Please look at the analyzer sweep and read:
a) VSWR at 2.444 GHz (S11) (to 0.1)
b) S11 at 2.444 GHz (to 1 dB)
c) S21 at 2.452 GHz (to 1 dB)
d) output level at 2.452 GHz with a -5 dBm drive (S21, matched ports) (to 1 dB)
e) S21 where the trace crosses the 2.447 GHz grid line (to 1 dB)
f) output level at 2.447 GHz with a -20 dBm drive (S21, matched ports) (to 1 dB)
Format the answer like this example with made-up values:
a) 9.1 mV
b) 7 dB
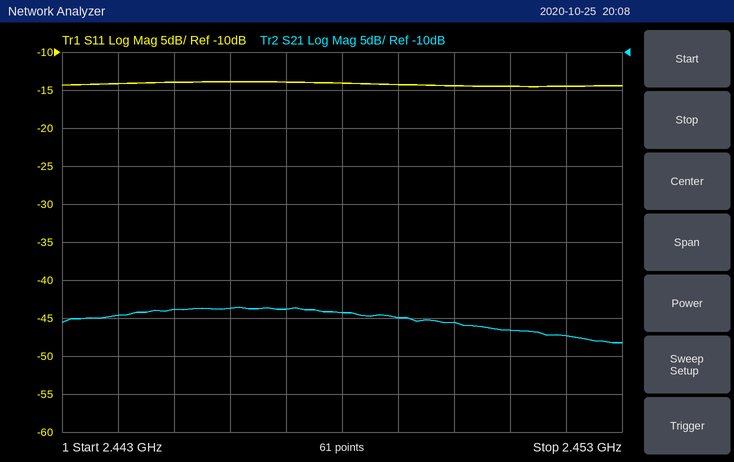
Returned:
a) 1.5
b) -14 dB
c) -47 dB
d) -52 dBm
e) -44 dB
f) -64 dBm
